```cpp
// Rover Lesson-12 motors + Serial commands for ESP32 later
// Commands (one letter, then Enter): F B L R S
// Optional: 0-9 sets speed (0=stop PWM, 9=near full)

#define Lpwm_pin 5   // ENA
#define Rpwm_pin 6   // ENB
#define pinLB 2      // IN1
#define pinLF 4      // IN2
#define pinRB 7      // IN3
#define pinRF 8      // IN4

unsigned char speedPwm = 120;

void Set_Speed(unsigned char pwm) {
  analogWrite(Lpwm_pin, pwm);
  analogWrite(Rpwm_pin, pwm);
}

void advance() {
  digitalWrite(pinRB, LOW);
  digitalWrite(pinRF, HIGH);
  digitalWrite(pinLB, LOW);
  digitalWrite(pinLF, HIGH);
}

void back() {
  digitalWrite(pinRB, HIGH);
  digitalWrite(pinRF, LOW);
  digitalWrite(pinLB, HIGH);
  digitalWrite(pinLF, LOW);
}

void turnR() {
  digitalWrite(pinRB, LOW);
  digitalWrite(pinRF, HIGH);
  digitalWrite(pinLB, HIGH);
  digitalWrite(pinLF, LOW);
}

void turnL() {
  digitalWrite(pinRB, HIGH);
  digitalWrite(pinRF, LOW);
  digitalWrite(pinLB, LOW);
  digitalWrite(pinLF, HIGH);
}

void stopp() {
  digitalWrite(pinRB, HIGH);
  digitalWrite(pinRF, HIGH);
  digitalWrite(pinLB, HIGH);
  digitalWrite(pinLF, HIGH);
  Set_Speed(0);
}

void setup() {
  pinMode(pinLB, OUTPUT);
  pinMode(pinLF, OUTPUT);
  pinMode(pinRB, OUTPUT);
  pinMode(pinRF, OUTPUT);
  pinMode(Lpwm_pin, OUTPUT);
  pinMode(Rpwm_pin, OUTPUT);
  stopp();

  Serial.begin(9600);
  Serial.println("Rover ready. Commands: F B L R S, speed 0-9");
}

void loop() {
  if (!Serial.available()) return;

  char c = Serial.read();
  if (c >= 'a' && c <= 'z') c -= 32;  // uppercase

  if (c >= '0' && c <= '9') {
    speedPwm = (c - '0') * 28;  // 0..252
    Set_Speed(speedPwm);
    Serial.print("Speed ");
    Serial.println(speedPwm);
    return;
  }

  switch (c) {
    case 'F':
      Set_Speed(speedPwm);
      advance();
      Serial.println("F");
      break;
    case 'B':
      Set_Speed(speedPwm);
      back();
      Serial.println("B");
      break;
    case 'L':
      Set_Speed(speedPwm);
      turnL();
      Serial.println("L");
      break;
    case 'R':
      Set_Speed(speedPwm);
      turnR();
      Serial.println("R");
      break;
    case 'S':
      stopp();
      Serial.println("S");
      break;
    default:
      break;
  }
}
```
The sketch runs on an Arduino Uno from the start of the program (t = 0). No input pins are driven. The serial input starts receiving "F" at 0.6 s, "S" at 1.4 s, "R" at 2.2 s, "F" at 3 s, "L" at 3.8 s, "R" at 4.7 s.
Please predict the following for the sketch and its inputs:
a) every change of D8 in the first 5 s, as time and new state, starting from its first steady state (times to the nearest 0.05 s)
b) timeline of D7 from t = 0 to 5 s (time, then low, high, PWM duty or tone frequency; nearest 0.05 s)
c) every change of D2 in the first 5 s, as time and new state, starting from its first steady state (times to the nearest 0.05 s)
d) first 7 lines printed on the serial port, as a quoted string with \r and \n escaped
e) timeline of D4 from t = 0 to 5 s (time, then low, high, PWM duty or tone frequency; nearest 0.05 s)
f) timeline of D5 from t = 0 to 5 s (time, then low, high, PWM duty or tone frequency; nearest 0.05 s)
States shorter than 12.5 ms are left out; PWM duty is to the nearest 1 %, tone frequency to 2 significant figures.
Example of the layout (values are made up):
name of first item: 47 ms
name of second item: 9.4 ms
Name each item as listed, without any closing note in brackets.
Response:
every change of D8 in the first 5 s, as time and new state, starting from its first steady state: 0 s high; 3.8 s low; 4.7 s high
timeline of D7 from t = 0 to 5 s: 0 s high; 0.6 s low; 1.4 s high; 2.2 s low; 3.8 s high; 4.7 s low
every change of D2 in the first 5 s, as time and new state, starting from its first steady state: 0 s high; 0.6 s low; 1.4 s high; 3 s low; 4.7 s high
first 7 lines printed on the serial port, as a quoted string with \r and \n escaped: "Rover ready. Commands: F B L R S, speed 0-9\r\nF\r\nS\r\nR\r\nF\r\nL\r\nR\r\n"
timeline of D4 from t = 0 to 5 s: 0 s high; 2.2 s low; 3 s high; 4.7 s low
timeline of D5 from t = 0 to 5 s: 0 s low; 0.6 s PWM 47 %; 1.4 s low; 2.2 s PWM 47 %
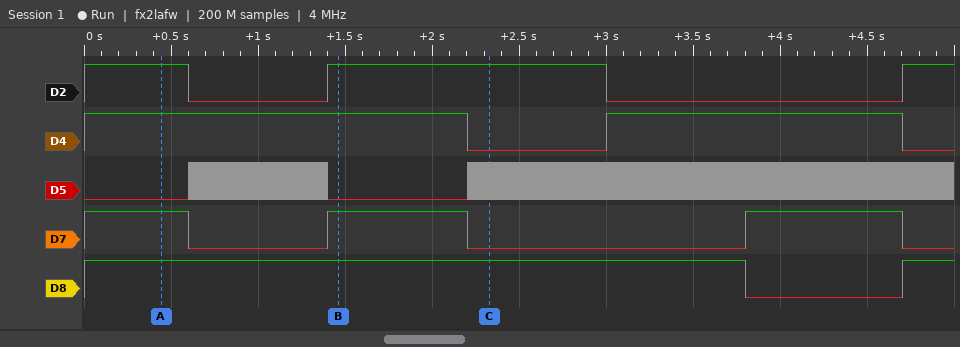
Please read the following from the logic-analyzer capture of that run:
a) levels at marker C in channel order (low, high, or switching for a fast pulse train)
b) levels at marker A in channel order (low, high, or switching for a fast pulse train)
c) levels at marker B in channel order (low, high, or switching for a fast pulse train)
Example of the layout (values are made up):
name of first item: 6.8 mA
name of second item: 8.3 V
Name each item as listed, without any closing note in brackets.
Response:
levels at marker C in channel order: D2 high, D4 low, D5 switching, D7 low, D8 high
levels at marker A in channel order: D2 high, D4 high, D5 low, D7 high, D8 high
levels at marker B in channel order: D2 high, D4 high, D5 low, D7 high, D8 high
